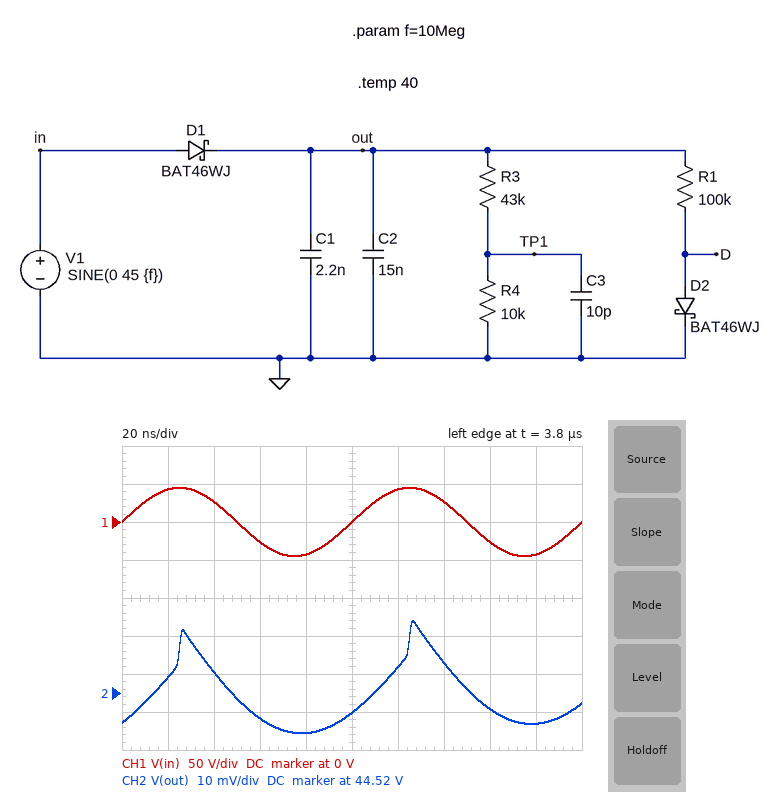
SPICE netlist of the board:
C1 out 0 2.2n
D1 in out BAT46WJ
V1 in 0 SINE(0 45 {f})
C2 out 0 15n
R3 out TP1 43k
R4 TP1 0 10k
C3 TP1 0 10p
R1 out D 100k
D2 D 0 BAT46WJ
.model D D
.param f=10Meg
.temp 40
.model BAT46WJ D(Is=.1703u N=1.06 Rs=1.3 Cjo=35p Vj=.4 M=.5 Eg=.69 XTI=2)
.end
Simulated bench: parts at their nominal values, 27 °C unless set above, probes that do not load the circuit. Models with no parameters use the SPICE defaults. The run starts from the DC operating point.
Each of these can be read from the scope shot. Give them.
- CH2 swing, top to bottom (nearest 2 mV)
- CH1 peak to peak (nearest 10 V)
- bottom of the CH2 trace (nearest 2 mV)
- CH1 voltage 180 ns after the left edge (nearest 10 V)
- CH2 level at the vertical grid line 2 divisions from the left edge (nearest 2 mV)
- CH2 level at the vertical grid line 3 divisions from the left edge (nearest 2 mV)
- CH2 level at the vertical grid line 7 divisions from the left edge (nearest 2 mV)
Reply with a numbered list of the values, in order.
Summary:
1. 30 mV
2. 90 V
3. 44.510 V
4. -40 V
5. 44.526 V
6. 44.514 V
7. 44.528 V
